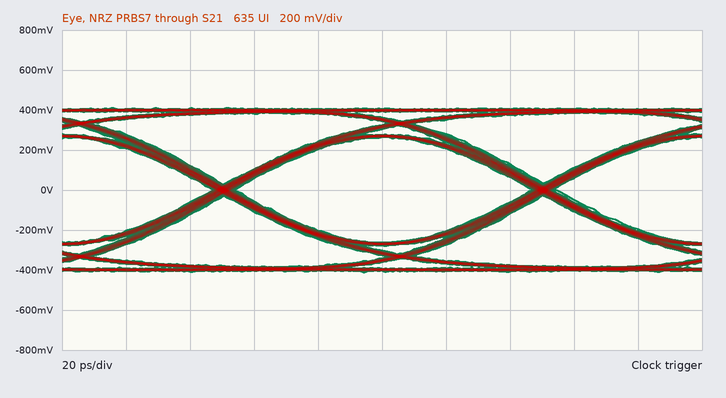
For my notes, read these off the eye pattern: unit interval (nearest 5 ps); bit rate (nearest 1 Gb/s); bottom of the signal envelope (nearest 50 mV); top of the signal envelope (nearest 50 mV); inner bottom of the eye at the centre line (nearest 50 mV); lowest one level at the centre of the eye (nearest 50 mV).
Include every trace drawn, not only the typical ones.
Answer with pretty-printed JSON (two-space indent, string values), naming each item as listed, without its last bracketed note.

{
  "unit interval": "100 ps",
  "bit rate": "10 Gb/s",
  "bottom of the signal envelope": "-400 mV",
  "top of the signal envelope": "400 mV",
  "inner bottom of the eye at the centre line": "-250 mV",
  "lowest one level at the centre of the eye": "250 mV"
}
